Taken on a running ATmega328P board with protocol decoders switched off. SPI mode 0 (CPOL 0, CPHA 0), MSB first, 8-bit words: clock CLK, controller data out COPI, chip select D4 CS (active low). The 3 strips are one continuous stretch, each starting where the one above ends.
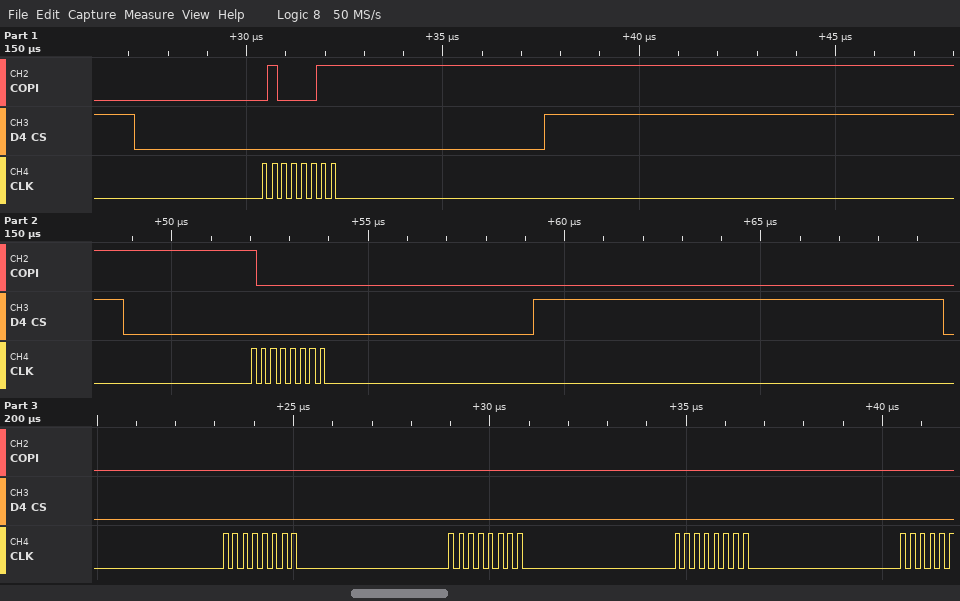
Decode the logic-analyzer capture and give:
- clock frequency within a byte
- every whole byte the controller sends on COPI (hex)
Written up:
4 MHz
0x43 0x80 0x00 0x00 0x00
